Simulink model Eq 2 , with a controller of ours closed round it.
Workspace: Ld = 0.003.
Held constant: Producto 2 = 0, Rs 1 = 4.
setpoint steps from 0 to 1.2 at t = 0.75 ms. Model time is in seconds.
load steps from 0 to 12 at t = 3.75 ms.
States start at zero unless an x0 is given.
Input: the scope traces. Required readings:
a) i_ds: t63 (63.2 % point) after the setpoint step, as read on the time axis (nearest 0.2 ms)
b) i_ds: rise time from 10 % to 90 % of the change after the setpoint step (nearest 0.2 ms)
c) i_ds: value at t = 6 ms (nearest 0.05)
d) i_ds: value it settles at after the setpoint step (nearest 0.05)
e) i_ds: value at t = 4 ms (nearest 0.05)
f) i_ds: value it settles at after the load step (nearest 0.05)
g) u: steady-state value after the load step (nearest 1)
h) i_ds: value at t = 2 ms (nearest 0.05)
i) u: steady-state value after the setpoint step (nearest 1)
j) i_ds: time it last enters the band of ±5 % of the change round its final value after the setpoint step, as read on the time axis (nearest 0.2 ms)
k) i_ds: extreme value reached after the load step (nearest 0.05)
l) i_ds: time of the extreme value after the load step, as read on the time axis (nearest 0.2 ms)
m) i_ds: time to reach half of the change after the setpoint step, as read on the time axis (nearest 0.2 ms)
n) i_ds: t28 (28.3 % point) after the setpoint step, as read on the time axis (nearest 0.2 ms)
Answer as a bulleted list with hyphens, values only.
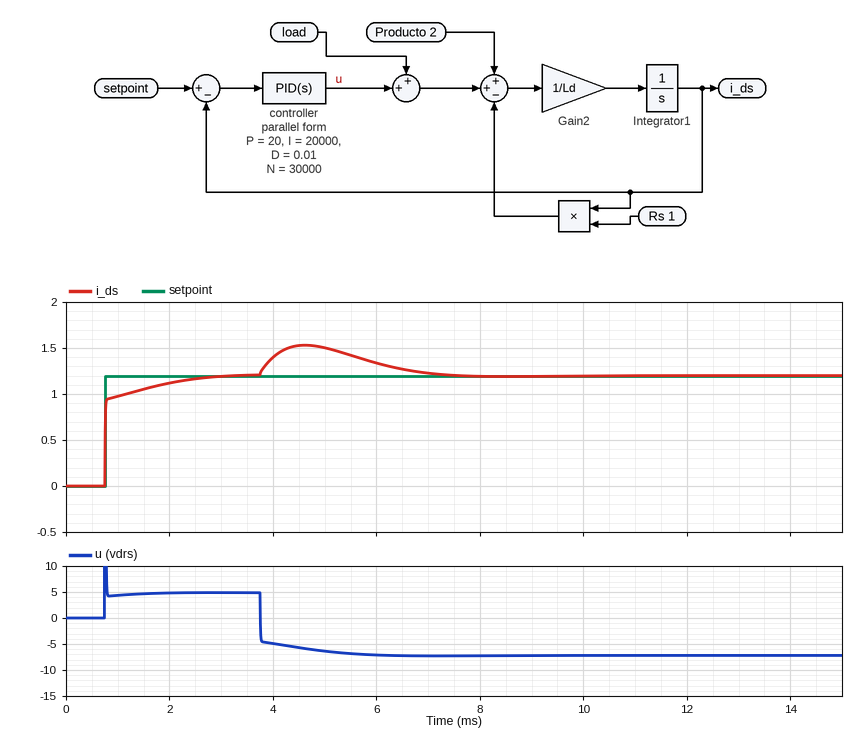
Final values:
- 0.8 ms
- 1.0 ms
- 1.35
- 1.20
- 1.40
- 1.20
- -7
- 1.10
- 5
- 2.2 ms
- 1.55
- 4.6 ms
- 0.8 ms
- 0.8 ms
